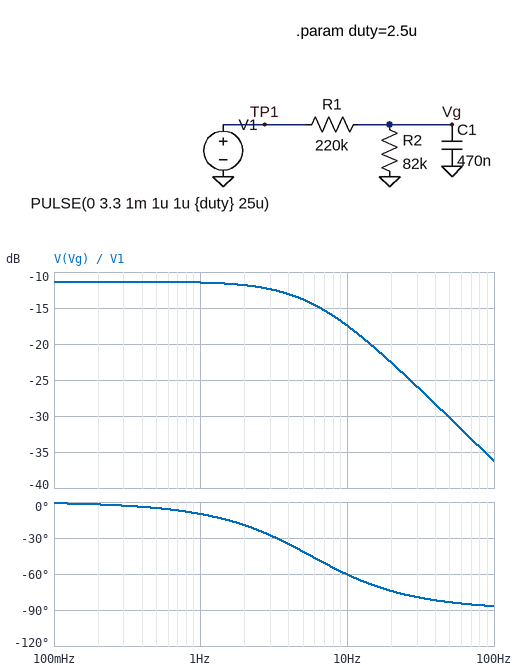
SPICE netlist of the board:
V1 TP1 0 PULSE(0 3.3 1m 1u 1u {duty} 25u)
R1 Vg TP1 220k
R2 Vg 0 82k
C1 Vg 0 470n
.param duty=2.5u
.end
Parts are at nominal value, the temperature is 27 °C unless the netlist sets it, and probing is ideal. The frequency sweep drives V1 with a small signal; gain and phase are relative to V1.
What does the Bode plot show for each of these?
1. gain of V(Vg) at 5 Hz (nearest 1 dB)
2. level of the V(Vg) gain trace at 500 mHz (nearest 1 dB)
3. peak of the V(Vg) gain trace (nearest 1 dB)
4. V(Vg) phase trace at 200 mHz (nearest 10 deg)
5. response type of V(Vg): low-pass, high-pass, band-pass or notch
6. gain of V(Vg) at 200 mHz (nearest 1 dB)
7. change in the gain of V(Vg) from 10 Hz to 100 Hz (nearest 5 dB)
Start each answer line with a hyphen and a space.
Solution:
- -14 dB
- -11 dB
- -11 dB
- 0 deg
- low-pass
- -11 dB
- -20 dB
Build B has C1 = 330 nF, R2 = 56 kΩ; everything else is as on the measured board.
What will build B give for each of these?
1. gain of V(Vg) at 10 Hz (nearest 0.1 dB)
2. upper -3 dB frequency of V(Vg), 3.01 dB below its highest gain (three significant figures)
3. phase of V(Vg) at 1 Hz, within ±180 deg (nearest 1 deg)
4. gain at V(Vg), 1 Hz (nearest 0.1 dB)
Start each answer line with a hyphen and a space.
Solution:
- -16.5 dB
- 10.8 Hz
- -5 deg
- -13.9 dB
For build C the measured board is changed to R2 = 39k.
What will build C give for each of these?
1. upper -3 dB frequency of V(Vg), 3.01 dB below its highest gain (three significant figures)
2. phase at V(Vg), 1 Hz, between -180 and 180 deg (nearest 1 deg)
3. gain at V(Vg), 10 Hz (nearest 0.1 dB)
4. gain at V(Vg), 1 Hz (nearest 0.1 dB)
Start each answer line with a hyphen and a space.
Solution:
- 10.2 Hz
- -6 deg
- -19.4 dB
- -16.5 dB
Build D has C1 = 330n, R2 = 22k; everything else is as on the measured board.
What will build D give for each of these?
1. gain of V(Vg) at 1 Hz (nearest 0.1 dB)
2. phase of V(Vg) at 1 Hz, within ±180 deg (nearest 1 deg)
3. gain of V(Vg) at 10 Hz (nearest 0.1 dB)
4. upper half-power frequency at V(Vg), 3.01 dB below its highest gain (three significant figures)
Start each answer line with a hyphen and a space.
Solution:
- -20.8 dB
- -2 deg
- -21.5 dB
- 24.1 Hz
